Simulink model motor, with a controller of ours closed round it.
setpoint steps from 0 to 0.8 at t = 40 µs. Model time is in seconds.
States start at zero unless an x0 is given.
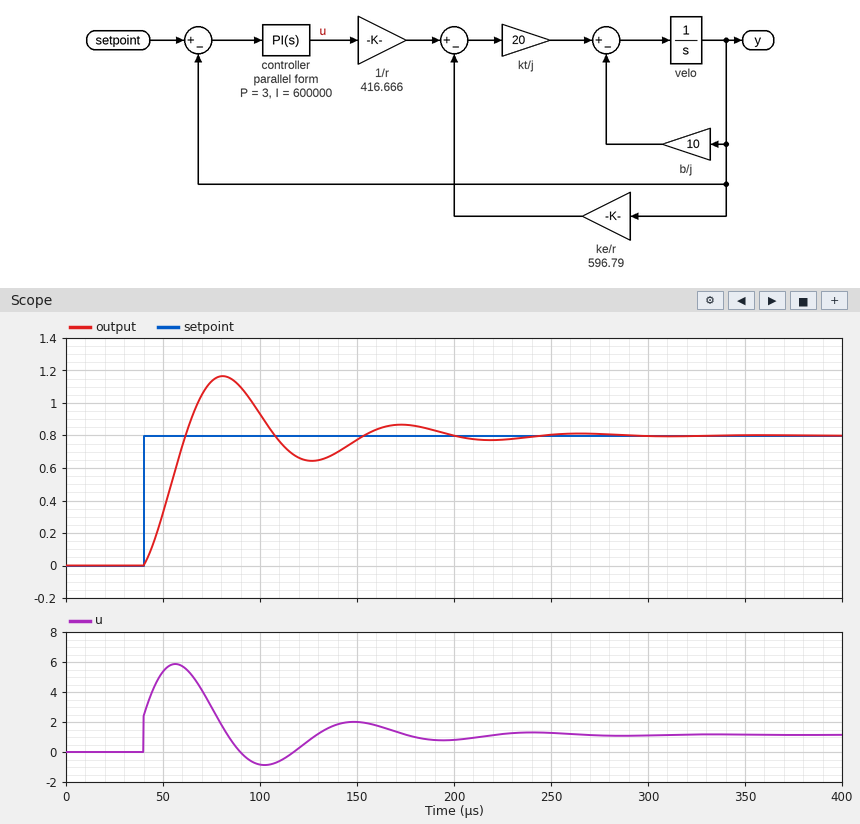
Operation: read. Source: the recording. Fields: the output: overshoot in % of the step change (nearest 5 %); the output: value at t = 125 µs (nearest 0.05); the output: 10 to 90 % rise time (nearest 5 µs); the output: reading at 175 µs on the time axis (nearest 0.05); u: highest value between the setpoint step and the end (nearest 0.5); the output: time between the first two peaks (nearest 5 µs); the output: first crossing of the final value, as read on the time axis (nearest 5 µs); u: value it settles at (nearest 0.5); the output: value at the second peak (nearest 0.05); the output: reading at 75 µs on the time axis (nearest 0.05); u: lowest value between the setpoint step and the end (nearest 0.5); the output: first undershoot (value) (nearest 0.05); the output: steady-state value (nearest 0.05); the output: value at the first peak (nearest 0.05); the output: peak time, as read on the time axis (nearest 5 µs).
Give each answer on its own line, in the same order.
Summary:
45 %
0.65
15 µs
0.85
6.0
90 µs
60 µs
1.0
0.85
1.15
-1.0
0.65
0.80
1.15
80 µs
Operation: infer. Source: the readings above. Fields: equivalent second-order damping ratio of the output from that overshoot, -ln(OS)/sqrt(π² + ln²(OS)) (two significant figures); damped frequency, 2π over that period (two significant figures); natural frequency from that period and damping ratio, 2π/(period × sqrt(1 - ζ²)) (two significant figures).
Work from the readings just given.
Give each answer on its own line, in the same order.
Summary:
0.25
0.070 rad/µs
0.072 rad/µs
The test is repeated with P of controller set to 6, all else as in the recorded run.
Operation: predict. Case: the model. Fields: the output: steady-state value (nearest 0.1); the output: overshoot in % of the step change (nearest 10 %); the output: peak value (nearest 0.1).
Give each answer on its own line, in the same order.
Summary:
0.8
30 %
1.0
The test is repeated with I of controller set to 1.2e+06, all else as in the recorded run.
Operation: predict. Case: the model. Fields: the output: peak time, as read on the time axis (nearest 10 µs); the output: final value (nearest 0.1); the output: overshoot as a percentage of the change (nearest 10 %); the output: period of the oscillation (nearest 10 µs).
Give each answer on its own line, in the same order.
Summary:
70 µs
0.8
60 %
60 µs
